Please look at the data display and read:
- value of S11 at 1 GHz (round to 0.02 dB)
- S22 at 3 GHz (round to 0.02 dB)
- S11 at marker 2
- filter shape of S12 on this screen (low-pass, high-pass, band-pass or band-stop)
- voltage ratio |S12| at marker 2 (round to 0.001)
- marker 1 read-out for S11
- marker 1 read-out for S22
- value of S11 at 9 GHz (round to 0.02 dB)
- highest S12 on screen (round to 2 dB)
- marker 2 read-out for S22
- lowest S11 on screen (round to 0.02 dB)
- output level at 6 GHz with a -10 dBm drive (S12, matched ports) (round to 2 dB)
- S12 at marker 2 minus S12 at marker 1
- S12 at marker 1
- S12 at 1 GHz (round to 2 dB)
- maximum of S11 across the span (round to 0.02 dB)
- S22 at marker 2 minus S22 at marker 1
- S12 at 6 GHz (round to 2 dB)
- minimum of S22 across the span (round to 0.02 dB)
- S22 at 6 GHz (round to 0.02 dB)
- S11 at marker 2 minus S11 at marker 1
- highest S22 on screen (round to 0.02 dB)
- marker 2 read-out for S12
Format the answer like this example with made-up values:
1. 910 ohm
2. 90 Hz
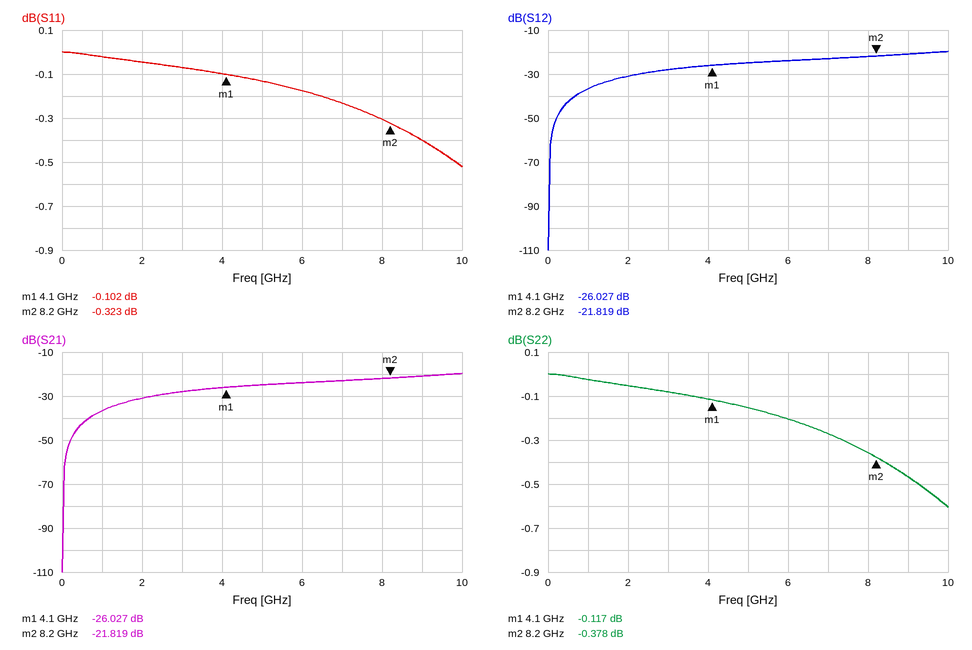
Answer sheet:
1. -0.02 dB
2. -0.08 dB
3. -0.323 dB
4. high-pass
5. 0.081
6. -0.102 dB
7. -0.117 dB
8. -0.40 dB
9. -20 dB
10. -0.378 dB
11. -0.52 dB
12. -34 dBm
13. 4.208 dB
14. -26.027 dB
15. -36 dB
16. 0.00 dB
17. -0.261 dB
18. -24 dB
19. -0.60 dB
20. -0.20 dB
21. -0.221 dB
22. 0.00 dB
23. -21.819 dB
